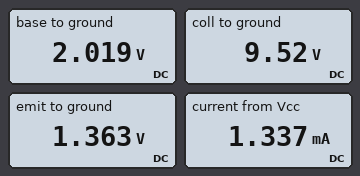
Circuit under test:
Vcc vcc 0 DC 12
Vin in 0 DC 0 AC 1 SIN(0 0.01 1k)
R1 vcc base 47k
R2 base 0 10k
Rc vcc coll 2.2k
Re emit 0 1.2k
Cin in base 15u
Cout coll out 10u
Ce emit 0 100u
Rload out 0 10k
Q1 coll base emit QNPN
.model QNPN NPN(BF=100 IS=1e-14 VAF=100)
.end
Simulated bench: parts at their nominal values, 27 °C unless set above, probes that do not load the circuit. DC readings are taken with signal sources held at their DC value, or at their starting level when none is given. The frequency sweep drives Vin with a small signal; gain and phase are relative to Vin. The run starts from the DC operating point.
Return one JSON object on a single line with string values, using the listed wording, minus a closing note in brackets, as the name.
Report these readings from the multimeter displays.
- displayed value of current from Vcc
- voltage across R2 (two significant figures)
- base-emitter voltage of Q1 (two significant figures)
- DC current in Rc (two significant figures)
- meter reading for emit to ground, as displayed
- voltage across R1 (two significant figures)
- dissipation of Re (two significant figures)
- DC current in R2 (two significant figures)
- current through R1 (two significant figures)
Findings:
{"displayed value of current from Vcc": "1.337 mA", "voltage across R2": "2.0 V", "base-emitter voltage of Q1": "660 mV", "DC current in Rc": "1.1 mA", "meter reading for emit to ground, as displayed": "1.363 V", "voltage across R1": "10 V", "dissipation of Re": "1.5 mW", "DC current in R2": "200 µA", "current through R1": "210 µA"}
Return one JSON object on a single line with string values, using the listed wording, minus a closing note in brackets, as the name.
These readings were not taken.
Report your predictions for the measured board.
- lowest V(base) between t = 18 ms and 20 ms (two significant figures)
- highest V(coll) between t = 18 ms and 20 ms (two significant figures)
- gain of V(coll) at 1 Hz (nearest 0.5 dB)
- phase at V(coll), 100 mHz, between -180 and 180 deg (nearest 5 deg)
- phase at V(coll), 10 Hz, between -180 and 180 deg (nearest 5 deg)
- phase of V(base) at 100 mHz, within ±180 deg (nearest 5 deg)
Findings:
{"lowest V(base) between t = 18 ms and 20 ms": "2.0 V", "highest V(coll) between t = 18 ms and 20 ms": "10 V", "gain of V(coll) at 1 Hz": "1.5 dB", "phase at V(coll), 100 mHz, between -180 and 180 deg": "-90 deg", "phase at V(coll), 10 Hz, between -180 and 180 deg": "-100 deg", "phase of V(base) at 100 mHz, within ±180 deg": "85 deg"}
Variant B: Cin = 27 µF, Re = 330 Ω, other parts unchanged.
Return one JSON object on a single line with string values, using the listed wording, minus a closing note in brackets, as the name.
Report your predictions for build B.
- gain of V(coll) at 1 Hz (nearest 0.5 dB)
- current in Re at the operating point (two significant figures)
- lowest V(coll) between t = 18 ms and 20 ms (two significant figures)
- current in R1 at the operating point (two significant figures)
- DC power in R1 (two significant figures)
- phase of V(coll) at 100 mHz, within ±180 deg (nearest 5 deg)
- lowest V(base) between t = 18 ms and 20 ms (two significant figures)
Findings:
{"gain of V(coll) at 1 Hz": "13.0 dB", "current in Re at the operating point": "3.5 mA", "lowest V(coll) between t = 18 ms and 20 ms": "2.1 V", "current in R1 at the operating point": "220 µA", "DC power in R1": "2.2 mW", "phase of V(coll) at 100 mHz, within ±180 deg": "-95 deg", "lowest V(base) between t = 18 ms and 20 ms": "1.8 V"}
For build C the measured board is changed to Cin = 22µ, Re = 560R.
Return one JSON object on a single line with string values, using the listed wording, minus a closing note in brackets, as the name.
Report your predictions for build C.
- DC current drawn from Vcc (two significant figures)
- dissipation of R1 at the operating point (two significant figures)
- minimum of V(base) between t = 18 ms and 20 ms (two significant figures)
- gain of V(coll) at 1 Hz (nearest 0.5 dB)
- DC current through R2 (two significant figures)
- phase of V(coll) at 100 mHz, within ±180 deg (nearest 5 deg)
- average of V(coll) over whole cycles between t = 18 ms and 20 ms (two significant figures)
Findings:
{"DC current drawn from Vcc": "2.4 mA", "dissipation of R1 at the operating point": "2.2 mW", "minimum of V(base) between t = 18 ms and 20 ms": "1.9 V", "gain of V(coll) at 1 Hz": "8.5 dB", "DC current through R2": "190 µA", "phase of V(coll) at 100 mHz, within ±180 deg": "-95 deg", "average of V(coll) over whole cycles between t = 18 ms and 20 ms": "7.1 V"}
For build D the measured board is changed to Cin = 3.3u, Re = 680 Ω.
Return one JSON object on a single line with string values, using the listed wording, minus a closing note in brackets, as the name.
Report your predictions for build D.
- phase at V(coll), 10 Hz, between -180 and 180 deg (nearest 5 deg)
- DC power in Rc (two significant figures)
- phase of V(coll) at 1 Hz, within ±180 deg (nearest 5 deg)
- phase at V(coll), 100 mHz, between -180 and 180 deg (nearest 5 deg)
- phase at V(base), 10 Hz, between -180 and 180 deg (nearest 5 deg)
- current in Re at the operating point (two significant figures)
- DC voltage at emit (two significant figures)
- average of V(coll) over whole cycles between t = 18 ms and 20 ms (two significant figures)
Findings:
{"phase at V(coll), 10 Hz, between -180 and 180 deg": "-80 deg", "DC power in Rc": "7.8 mW", "phase of V(coll) at 1 Hz, within ±180 deg": "-85 deg", "phase at V(coll), 100 mHz, between -180 and 180 deg": "-90 deg", "phase at V(base), 10 Hz, between -180 and 180 deg": "30 deg", "current in Re at the operating point": "1.9 mA", "DC voltage at emit": "1.3 V", "average of V(coll) over whole cycles between t = 18 ms and 20 ms": "7.9 V"}
